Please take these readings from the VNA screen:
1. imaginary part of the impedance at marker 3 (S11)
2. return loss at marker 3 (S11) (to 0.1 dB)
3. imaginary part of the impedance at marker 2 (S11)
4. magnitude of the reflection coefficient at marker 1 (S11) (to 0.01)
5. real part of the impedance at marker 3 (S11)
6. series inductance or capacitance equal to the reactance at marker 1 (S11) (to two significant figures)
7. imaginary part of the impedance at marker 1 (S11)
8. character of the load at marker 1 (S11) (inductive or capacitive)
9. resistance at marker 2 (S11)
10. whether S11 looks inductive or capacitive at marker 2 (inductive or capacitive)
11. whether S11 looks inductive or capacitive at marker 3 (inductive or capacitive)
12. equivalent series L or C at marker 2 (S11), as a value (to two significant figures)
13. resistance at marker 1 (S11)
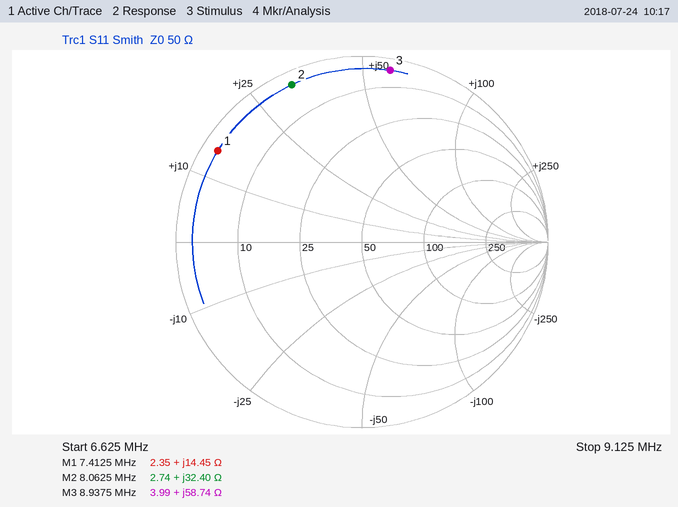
+58.74 Ω
0.6 dB
+32.40 Ω
0.92
3.99 Ω
310 nH
+14.45 Ω
inductive
2.74 Ω
inductive
inductive
640 nH
2.35 Ω
